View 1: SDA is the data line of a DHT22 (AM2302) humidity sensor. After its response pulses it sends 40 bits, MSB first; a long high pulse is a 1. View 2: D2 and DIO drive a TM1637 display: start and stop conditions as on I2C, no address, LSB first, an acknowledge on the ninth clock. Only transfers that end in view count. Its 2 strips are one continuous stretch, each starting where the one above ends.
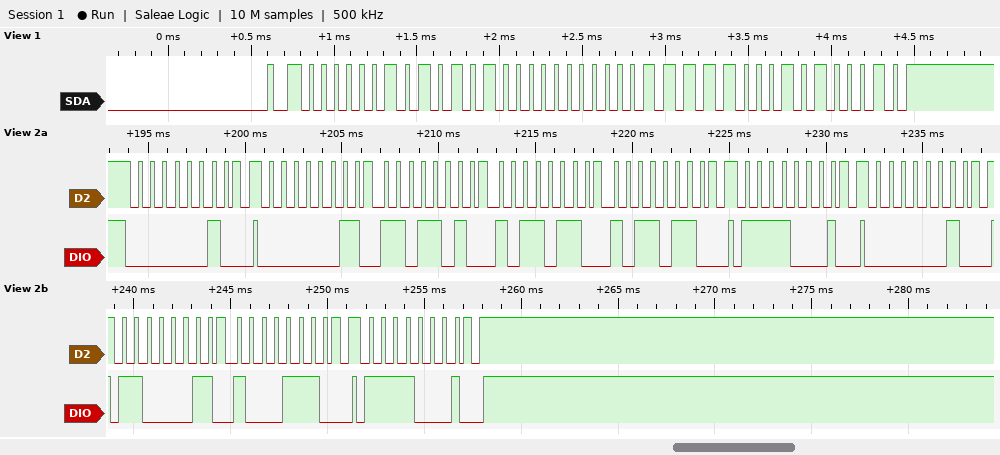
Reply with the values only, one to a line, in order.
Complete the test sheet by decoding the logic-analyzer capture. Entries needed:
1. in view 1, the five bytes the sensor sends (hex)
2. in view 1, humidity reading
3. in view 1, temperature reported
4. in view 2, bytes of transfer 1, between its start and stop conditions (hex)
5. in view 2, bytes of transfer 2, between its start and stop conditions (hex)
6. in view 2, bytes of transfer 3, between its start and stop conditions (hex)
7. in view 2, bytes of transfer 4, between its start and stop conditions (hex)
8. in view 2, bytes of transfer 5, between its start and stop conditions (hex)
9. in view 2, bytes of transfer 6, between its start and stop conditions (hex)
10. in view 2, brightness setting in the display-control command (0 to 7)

02 A8 00 F8 A2
68.0 %
24.8 °C
40
C0 5B 6D 6D
8F
40
C3 71
8F
7
